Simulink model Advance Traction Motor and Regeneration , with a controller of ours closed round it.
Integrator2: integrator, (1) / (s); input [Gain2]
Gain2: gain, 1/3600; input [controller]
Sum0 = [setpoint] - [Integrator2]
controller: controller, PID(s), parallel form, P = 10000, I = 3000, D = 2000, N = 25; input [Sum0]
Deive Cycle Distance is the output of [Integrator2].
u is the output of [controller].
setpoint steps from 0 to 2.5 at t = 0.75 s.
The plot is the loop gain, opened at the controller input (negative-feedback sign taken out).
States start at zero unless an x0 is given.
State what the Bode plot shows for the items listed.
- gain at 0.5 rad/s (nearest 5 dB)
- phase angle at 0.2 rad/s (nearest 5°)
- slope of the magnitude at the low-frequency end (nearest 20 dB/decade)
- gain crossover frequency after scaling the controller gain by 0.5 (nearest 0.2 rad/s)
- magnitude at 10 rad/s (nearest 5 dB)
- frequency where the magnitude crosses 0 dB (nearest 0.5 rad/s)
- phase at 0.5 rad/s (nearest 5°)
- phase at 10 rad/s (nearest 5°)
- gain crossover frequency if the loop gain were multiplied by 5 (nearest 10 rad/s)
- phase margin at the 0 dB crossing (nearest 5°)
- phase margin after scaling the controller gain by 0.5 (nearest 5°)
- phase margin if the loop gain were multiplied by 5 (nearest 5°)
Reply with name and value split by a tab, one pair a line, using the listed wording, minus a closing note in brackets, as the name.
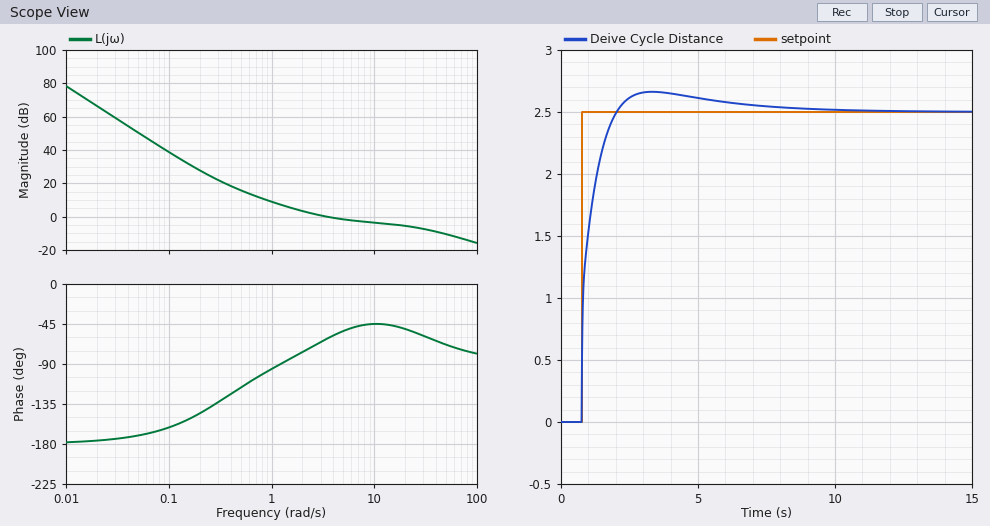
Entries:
gain at 0.5 rad/s	15 dB
phase angle at 0.2 rad/s	-145°
slope of the magnitude at the low-frequency end	-40 dB/decade
gain crossover frequency after scaling the controller gain by 0.5	1.4 rad/s
magnitude at 10 rad/s	-5 dB
frequency where the magnitude crosses 0 dB	3.5 rad/s
phase at 0.5 rad/s	-115°
phase at 10 rad/s	-45°
gain crossover frequency if the loop gain were multiplied by 5	80 rad/s
phase margin at the 0 dB crossing	120°
phase margin after scaling the controller gain by 0.5	95°
phase margin if the loop gain were multiplied by 5	105°
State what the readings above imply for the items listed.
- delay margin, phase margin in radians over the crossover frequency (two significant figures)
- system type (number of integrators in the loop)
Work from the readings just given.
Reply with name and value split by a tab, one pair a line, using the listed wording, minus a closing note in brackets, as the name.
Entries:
delay margin, phase margin in radians over the crossover frequency	0.60 s
system type	2
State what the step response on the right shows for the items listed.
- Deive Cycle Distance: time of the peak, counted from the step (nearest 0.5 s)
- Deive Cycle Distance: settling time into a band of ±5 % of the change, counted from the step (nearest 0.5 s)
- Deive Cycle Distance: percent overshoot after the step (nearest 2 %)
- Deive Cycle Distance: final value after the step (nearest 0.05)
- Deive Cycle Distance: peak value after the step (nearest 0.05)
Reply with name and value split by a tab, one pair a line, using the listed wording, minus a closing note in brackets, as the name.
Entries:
Deive Cycle Distance: time of the peak, counted from the step	2.5 s
Deive Cycle Distance: settling time into a band of ±5 % of the change, counted from the step	4.0 s
Deive Cycle Distance: percent overshoot after the step	6 %
Deive Cycle Distance: final value after the step	2.50
Deive Cycle Distance: peak value after the step	2.65
